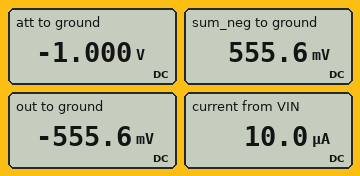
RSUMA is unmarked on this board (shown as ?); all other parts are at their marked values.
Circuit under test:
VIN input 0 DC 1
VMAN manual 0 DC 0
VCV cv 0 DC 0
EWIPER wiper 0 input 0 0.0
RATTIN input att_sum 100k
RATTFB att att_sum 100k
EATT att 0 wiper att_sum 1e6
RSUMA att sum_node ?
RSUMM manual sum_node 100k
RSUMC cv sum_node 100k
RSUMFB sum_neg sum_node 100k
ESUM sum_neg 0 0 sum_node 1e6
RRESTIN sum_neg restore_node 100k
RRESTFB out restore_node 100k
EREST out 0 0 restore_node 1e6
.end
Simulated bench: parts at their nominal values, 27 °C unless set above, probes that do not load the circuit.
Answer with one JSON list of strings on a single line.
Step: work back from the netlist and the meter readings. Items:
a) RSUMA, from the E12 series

["180 kΩ"]
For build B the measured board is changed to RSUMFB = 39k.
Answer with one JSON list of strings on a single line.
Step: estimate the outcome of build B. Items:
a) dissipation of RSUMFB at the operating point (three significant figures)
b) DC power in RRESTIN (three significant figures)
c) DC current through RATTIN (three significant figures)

["1.20 µW", "469 nW", "10.0 µA"]
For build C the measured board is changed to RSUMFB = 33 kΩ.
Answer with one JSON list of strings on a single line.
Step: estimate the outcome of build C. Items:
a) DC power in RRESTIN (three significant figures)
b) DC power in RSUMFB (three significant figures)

["336 nW", "1.02 µW"]
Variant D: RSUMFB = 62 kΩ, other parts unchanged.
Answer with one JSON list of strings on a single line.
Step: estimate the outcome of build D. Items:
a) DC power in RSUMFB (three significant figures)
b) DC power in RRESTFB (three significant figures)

["1.91 µW", "1.19 µW"]
